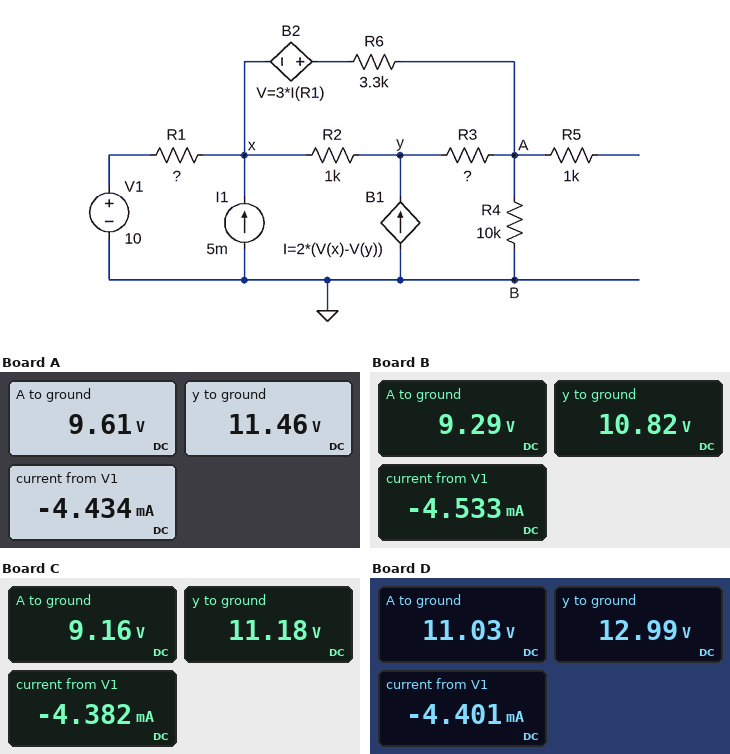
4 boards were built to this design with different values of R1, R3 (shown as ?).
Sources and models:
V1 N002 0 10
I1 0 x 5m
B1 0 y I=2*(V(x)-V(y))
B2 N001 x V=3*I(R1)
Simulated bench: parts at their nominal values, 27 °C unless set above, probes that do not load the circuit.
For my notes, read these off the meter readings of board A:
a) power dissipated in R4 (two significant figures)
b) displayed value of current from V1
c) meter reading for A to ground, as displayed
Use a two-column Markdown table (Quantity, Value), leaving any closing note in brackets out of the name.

| Quantity | Value |
|---|---|
| power dissipated in R4 | 9.2 mW |
| displayed value of current from V1 | -4.434 mA |
| meter reading for A to ground, as displayed | 9.61 V |
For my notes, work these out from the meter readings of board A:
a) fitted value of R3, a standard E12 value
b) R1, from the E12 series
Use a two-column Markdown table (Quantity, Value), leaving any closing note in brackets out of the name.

| Quantity | Value |
|---|---|
| fitted value of R3, a standard E12 value | 4.7 kΩ |
| R1, from the E12 series | 330 Ω |
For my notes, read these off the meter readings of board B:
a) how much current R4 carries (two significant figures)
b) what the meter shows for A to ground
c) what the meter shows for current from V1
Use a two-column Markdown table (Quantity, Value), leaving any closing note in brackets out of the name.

| Quantity | Value |
|---|---|
| how much current R4 carries | 930 µA |
| what the meter shows for A to ground | 9.29 V |
| what the meter shows for current from V1 | -4.533 mA |
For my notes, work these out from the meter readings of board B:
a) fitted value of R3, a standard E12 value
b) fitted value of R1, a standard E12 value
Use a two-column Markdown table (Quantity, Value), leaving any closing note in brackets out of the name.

| Quantity | Value |
|---|---|
| fitted value of R3, a standard E12 value | 3.3 kΩ |
| fitted value of R1, a standard E12 value | 180 Ω |
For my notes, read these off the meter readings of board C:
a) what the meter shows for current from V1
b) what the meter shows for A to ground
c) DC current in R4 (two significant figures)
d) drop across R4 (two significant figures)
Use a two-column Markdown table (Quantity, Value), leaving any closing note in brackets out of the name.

| Quantity | Value |
|---|---|
| what the meter shows for current from V1 | -4.382 mA |
| what the meter shows for A to ground | 9.16 V |
| DC current in R4 | 920 µA |
| drop across R4 | 9.2 V |
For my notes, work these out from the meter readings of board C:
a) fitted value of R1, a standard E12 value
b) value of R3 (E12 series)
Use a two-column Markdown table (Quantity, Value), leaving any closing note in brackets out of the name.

| Quantity | Value |
|---|---|
| fitted value of R1, a standard E12 value | 270 Ω |
| value of R3 | 6.8 kΩ |
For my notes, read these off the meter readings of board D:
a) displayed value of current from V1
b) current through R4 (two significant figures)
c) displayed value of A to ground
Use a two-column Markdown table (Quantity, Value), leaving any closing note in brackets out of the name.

| Quantity | Value |
|---|---|
| displayed value of current from V1 | -4.401 mA |
| current through R4 | 1.1 mA |
| displayed value of A to ground | 11.03 V |
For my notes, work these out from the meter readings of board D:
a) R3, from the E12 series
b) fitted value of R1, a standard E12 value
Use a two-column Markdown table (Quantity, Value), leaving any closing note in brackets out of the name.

| Quantity | Value |
|---|---|
| R3, from the E12 series | 3.9 kΩ |
| fitted value of R1, a standard E12 value | 680 Ω |
